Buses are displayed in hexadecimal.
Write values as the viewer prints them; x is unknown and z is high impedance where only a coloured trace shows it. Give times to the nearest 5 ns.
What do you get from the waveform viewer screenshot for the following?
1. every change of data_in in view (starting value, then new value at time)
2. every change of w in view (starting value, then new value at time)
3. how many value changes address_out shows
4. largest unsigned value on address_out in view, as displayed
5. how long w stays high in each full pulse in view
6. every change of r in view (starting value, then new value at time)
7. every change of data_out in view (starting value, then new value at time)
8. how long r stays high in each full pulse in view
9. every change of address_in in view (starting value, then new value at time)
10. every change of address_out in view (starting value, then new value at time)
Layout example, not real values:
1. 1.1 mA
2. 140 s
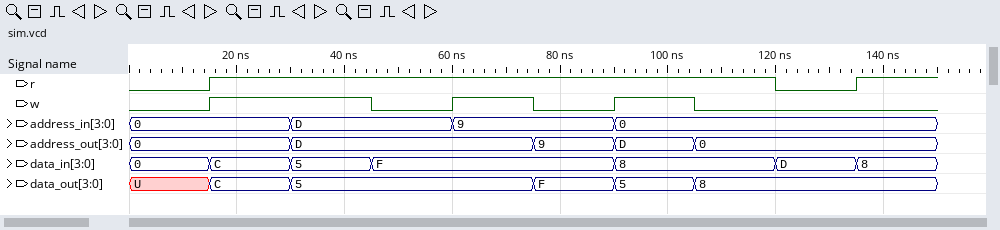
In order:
1. 0, C at 15 ns, 5 at 30 ns, F at 45 ns, 8 at 90 ns, D at 120 ns, 8 at 135 ns
2. 0, 1 at 15 ns, 0 at 45 ns, 1 at 60 ns, 0 at 75 ns, 1 at 90 ns, 0 at 105 ns
3. 4
4. D
5. 30 ns, 15 ns, 15 ns
6. 0, 1 at 15 ns, 0 at 120 ns, 1 at 135 ns
7. U, C at 15 ns, 5 at 30 ns, F at 75 ns, 5 at 90 ns, 8 at 105 ns
8. 105 ns
9. 0, D at 30 ns, 9 at 60 ns, 0 at 90 ns
10. 0, D at 30 ns, 9 at 75 ns, D at 90 ns, 0 at 105 ns
